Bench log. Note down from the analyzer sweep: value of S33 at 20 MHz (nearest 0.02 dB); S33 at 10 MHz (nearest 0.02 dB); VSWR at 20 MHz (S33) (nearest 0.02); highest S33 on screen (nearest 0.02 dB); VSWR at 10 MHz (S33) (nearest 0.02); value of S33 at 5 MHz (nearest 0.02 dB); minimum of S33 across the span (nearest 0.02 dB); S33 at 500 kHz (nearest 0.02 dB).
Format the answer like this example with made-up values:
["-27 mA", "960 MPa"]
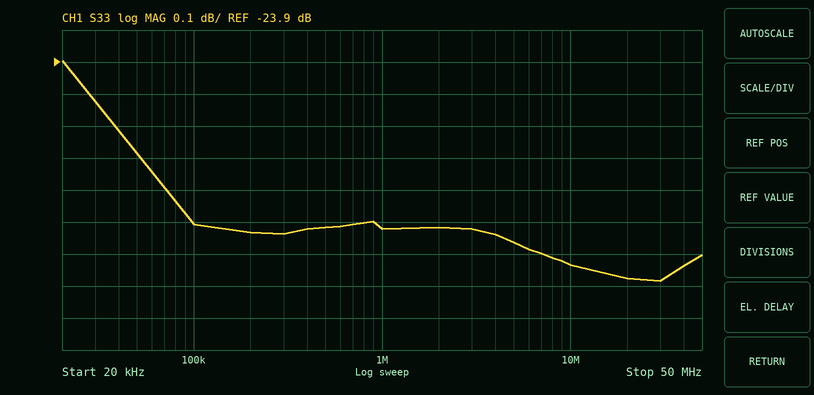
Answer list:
["-24.58 dB", "-24.54 dB", "1.12", "-23.90 dB", "1.12", "-24.46 dB", "-24.58 dB", "-24.42 dB"]
